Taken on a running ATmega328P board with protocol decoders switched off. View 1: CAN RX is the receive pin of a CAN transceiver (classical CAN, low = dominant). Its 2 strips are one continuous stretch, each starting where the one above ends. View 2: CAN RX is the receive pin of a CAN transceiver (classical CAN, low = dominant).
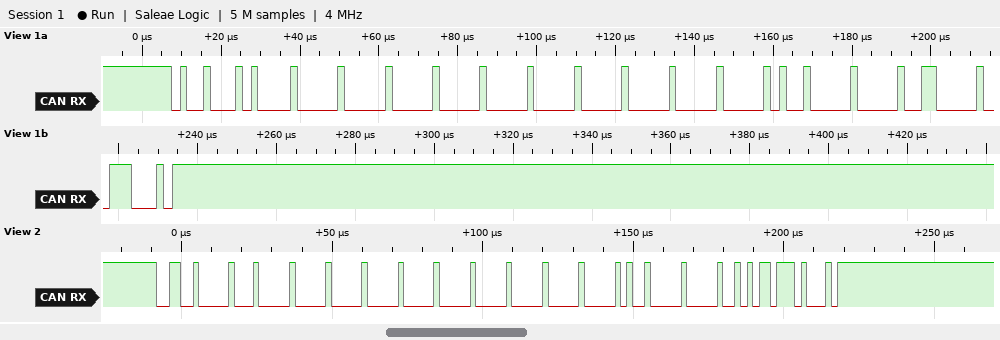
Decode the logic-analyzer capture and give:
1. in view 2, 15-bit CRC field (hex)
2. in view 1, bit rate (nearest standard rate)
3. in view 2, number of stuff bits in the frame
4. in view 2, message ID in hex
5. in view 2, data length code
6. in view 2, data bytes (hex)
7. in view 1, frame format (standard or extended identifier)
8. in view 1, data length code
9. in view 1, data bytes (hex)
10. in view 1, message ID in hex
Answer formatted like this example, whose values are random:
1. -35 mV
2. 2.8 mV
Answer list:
1. 0x56E8
2. 500 kbit/s
3. 13
4. 0x320
5. 8
6. 00 00 00 00 00 00 90 00
7. standard
8. 8
9. 00 00 00 00 00 00 90 00
10. 0x48A
